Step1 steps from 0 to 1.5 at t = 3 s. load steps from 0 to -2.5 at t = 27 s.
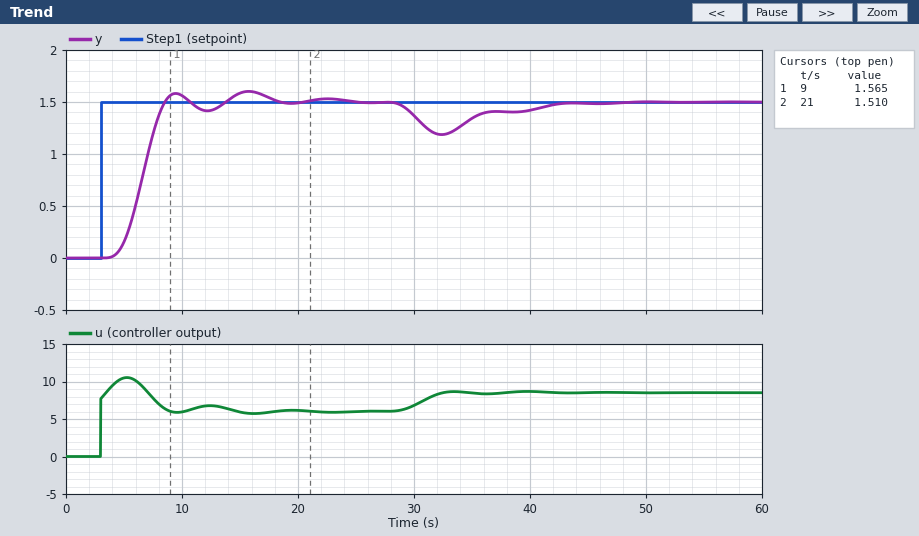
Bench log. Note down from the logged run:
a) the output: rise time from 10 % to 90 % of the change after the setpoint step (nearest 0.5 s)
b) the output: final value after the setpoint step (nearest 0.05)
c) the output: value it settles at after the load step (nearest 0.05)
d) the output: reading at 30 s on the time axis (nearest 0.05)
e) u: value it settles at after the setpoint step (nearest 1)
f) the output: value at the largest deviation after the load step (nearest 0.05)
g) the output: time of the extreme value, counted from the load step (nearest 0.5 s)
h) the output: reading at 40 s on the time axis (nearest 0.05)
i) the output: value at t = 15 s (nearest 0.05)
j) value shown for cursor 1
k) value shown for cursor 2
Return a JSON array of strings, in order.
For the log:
["3.0 s", "1.50", "1.50", "1.35", "6", "1.20", "5.5 s", "1.40", "1.60", "1.565", "1.510"]
